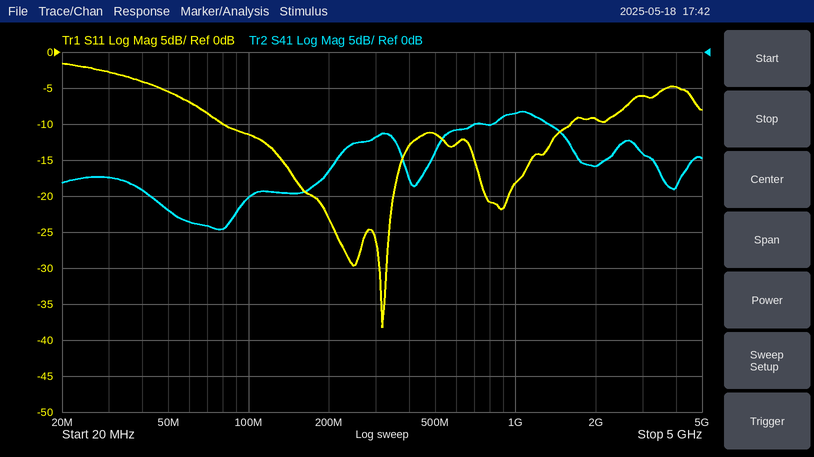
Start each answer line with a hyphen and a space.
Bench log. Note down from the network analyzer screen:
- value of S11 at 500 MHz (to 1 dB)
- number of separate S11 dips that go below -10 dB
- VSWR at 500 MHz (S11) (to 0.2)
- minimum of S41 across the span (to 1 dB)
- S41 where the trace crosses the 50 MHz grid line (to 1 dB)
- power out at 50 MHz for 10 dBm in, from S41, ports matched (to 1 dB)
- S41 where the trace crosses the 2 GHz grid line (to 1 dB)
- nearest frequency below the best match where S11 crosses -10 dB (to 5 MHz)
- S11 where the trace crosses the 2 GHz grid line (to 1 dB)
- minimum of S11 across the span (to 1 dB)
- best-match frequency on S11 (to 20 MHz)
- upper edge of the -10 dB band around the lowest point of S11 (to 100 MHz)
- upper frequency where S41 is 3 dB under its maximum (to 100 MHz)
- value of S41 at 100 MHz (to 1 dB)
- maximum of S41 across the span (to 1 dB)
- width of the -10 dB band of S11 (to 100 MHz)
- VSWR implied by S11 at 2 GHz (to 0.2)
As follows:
- -11 dB
- 3
- 1.8
- -25 dB
- -22 dB
- -12 dBm
- -16 dB
- 80 MHz
- -9 dB
- -38 dB
- 320 MHz
- 1.6 GHz
- 1.5 GHz
- -20 dB
- -8 dB
- 1.5 GHz
- 2.0
